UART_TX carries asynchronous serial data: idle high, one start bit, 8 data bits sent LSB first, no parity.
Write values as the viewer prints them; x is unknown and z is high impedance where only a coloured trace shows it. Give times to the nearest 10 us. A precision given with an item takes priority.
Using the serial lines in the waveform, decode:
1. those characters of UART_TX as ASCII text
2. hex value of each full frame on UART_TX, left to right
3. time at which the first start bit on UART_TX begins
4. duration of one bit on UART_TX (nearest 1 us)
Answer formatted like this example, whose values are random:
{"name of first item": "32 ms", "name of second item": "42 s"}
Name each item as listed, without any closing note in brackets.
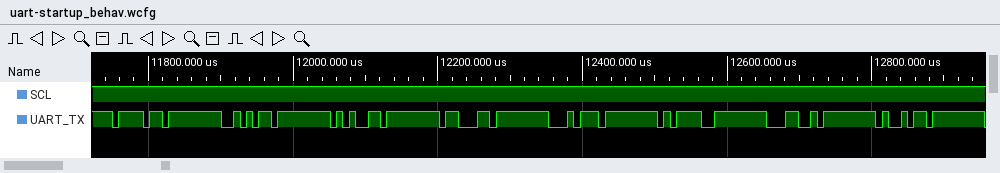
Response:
{"those characters of UART_TX as ASCII text": "\"oject=Li\"", "hex value of each full frame on UART_TX, left to right": "6F, 6A, 65, 63, 74, 3D, 4C, 69", "time at which the first start bit on UART_TX begins": "11750 us", "duration of one bit on UART_TX": "9 us"}
